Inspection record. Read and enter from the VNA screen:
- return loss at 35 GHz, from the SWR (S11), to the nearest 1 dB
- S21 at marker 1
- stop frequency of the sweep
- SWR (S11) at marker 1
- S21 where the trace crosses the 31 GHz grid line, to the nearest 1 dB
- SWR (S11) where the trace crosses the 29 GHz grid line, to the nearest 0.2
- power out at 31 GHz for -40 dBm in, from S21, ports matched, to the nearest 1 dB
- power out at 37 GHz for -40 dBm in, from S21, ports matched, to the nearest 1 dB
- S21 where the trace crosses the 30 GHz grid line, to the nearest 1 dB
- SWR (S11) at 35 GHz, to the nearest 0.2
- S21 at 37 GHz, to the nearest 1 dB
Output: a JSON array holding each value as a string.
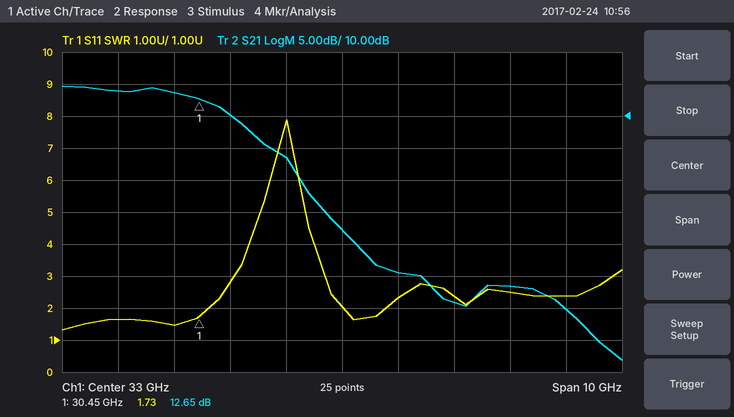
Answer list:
["8 dB", "12.65 dB", "38 GHz", "1.73", "10 dB", "1.6", "-30 dBm", "-60 dBm", "14 dB", "2.4", "-20 dB"]
